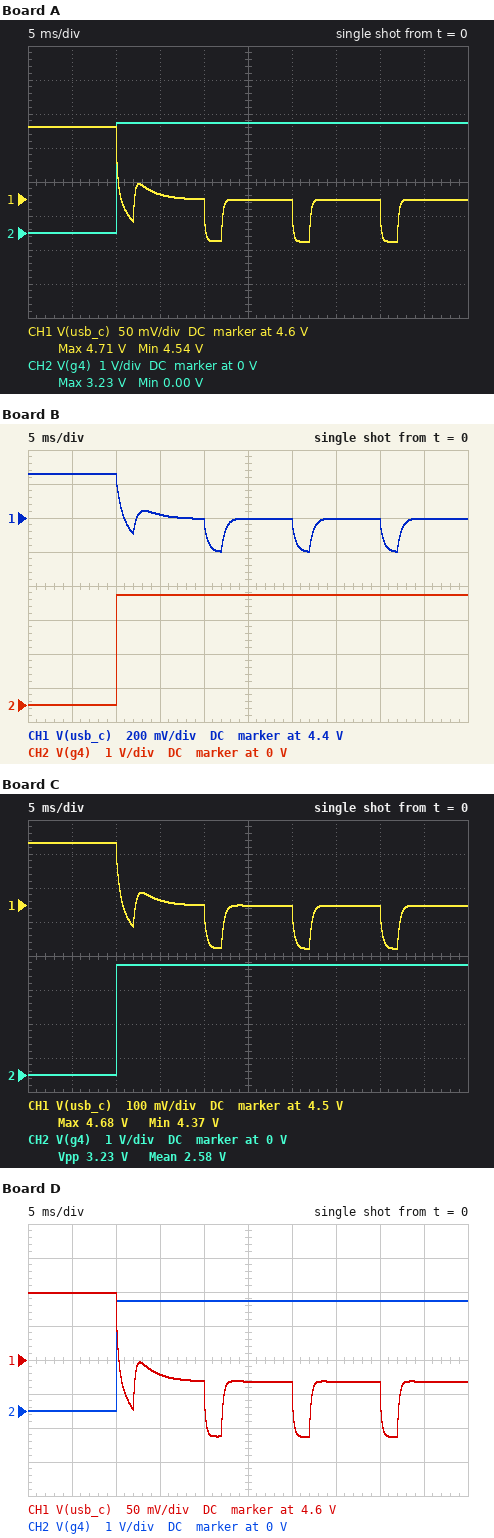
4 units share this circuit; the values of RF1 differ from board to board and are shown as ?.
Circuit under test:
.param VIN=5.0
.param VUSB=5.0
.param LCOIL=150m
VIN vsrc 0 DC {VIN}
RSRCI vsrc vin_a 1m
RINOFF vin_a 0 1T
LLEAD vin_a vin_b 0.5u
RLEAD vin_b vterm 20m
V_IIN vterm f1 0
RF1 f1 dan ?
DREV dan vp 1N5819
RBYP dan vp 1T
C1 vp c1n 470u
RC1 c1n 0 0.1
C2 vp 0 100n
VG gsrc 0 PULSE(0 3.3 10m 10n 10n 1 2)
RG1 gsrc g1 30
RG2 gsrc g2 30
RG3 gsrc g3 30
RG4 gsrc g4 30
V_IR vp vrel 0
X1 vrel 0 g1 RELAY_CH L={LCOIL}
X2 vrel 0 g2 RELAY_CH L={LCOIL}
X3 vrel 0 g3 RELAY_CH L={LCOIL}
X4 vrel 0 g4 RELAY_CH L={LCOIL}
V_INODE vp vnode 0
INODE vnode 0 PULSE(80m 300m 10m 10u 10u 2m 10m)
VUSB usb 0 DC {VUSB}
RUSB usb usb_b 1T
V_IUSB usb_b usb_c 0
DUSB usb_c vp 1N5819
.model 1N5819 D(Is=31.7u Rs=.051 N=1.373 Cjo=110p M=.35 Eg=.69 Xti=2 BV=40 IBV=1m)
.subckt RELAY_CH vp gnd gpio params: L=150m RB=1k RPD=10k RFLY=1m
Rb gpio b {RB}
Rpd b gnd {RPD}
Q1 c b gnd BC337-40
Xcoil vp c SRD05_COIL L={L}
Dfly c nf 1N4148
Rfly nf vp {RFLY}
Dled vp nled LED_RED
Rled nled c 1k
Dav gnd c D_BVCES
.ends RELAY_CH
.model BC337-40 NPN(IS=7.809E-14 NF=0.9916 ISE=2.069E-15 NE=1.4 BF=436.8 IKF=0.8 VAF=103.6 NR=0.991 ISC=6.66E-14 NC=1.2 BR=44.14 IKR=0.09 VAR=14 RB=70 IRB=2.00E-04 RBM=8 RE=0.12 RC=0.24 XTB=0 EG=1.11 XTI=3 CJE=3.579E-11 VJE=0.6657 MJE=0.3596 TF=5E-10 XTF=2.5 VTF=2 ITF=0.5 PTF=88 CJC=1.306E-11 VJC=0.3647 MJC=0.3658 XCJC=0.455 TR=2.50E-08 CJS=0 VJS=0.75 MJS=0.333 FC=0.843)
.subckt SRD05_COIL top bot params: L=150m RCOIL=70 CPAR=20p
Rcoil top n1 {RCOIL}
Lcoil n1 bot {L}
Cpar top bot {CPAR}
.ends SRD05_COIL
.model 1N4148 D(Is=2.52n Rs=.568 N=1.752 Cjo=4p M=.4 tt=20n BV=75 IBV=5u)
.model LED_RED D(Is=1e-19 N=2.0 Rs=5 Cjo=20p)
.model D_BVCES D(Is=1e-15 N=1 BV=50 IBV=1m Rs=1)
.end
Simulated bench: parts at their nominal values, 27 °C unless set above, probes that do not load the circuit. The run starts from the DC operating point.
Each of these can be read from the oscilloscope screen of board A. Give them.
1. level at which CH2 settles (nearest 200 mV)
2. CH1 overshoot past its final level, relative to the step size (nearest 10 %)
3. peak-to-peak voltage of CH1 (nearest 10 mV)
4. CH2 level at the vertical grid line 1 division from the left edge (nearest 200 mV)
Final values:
3.2 V
60 %
170 mV
0 V
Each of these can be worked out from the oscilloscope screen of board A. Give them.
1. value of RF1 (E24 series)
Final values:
0.13 Ω
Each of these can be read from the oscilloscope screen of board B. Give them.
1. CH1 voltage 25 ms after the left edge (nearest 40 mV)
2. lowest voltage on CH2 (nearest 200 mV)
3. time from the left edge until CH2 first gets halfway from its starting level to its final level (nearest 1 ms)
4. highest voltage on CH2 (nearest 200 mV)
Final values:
4.40 V
0 V
10 ms
3.2 V
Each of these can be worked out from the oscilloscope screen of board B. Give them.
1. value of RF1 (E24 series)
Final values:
0.75 Ω
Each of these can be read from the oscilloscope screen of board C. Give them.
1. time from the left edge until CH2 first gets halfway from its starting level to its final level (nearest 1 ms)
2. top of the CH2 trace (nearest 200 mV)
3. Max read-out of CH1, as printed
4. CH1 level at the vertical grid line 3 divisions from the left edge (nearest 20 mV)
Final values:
10 ms
3.2 V
4.68 V
4.52 V
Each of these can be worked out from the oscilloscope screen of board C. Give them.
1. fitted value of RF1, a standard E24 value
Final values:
0.43 Ω
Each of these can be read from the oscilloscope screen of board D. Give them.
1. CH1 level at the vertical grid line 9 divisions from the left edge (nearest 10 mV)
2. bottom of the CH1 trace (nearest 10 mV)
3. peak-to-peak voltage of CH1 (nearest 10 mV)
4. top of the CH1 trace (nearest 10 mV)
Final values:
4.57 V
4.49 V
210 mV
4.70 V
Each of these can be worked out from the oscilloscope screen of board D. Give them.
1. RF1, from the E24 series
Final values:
0.22 Ω
